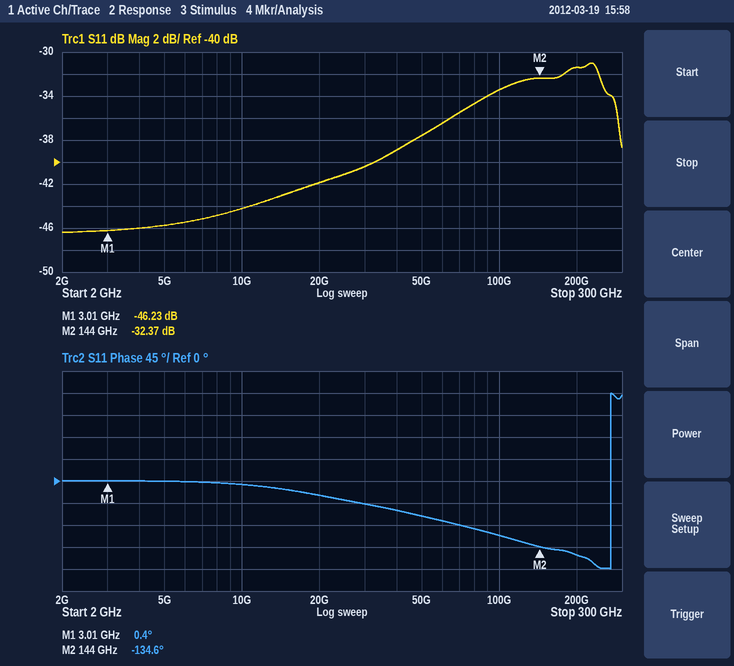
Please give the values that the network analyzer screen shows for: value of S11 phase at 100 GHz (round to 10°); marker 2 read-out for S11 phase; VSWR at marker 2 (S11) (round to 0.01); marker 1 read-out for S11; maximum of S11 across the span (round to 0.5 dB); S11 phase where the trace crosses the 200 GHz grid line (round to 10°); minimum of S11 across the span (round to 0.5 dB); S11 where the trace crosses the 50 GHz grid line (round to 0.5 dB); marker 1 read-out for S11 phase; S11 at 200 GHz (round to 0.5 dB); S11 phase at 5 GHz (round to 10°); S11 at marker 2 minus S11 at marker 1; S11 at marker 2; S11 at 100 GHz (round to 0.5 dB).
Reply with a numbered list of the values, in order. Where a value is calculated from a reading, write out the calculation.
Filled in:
1. -110°
2. -134.6°
3. (1 + 0.0241)/(1 − 0.0241) ≈ 1.05
4. -46.23 dB
5. -31.0 dB
6. -150°
7. -46.5 dB
8. -37.5 dB
9. 0.4°
10. -31.5 dB
11. 0°
12. -32.37 − (-46.23) = 13.86 dB
13. -32.37 dB
14. -33.5 dB
